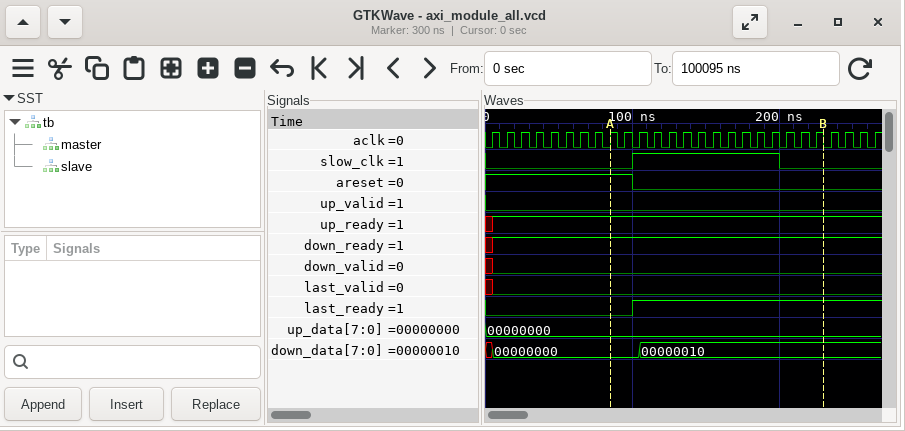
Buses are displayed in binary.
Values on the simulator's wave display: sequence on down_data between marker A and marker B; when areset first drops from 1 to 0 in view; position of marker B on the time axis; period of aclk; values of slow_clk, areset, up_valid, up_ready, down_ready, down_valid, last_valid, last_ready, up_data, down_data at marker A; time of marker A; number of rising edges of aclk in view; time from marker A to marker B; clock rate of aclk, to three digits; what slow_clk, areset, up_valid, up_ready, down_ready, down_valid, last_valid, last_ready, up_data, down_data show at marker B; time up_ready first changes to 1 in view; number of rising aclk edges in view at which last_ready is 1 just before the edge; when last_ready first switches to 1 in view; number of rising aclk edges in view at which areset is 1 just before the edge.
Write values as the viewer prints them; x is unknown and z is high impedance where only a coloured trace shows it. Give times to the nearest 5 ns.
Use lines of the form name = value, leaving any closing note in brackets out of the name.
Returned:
sequence on down_data between marker A and marker B = 00000000, 00000010
when areset first drops from 1 to 0 in view = 100 ns
position of marker B on the time axis = 230 ns
period of aclk = 10 ns
values of slow_clk, areset, up_valid, up_ready, down_ready, down_valid, last_valid, last_ready, up_data, down_data at marker A = slow_clk=0, areset=1, up_valid=0, up_ready=1, down_ready=1, down_valid=0, last_valid=0, last_ready=0, up_data=00000000, down_data=00000000
time of marker A = 85 ns
number of rising edges of aclk in view = 27
time from marker A to marker B = 145 ns
clock rate of aclk, to three digits = 100 MHz
what slow_clk, areset, up_valid, up_ready, down_ready, down_valid, last_valid, last_ready, up_data, down_data show at marker B = slow_clk=0, areset=0, up_valid=0, up_ready=1, down_ready=1, down_valid=0, last_valid=0, last_ready=1, up_data=00000000, down_data=00000010
time up_ready first changes to 1 in view = 5 ns
number of rising aclk edges in view at which last_ready is 1 just before the edge = 17
when last_ready first switches to 1 in view = 100 ns
number of rising aclk edges in view at which areset is 1 just before the edge = 10
